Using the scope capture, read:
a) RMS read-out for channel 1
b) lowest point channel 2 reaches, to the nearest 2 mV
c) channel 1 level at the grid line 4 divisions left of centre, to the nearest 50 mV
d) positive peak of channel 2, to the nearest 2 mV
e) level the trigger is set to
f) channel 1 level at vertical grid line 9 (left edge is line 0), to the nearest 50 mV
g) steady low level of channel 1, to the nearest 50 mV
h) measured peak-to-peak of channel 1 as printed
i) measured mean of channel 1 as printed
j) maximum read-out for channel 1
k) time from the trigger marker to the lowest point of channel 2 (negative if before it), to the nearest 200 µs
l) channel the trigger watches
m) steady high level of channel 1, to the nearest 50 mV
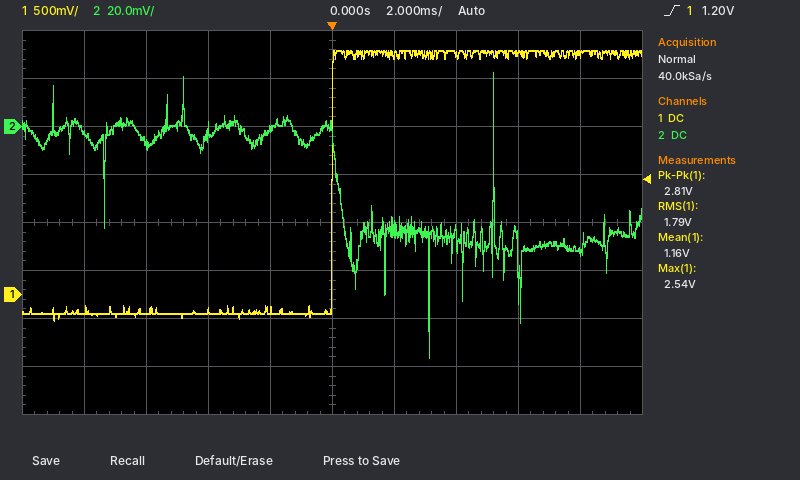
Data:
1.79 V
-96 mV
-150 mV
22 mV
1.20 V
2.50 V
-200 mV
2.81 V
1.16 V
2.54 V
+3.2 ms
channel 1
2.55 V
